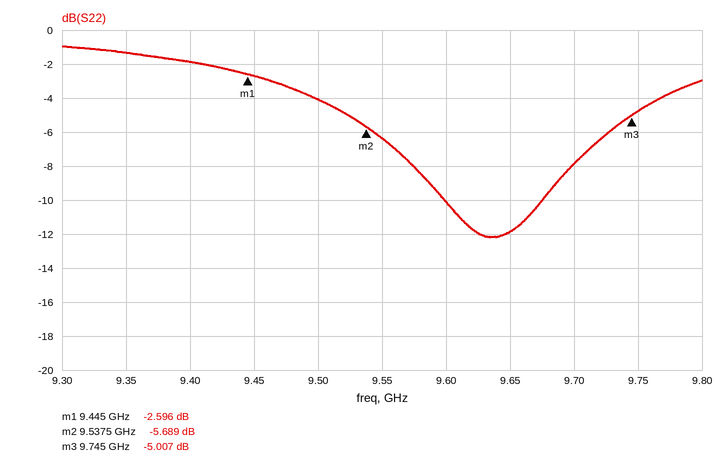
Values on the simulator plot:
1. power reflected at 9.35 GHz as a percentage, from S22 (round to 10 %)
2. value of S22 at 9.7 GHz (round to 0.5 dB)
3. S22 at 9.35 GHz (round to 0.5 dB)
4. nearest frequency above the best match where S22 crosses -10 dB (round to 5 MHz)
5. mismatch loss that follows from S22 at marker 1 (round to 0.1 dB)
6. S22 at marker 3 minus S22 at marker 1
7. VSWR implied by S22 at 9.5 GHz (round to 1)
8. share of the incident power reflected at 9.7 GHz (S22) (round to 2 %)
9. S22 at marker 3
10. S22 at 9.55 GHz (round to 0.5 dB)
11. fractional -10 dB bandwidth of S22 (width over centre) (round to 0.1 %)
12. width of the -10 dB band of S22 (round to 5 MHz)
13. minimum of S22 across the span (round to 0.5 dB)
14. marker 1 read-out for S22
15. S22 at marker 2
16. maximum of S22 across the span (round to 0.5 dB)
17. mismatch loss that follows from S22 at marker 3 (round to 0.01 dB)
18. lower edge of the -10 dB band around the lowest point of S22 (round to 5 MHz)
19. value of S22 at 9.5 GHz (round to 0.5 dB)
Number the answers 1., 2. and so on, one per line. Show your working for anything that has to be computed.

1. 10^(-1.5/10) ≈ 70.8 %, so 70 % to the nearest 10 %
2. -8.0 dB
3. -1.5 dB
4. 9.675 GHz
5. −10 log10(1 − 10^(-2.596/10)) ≈ 3.5 dB
6. -5.007 − (-2.596) = -2.411 dB
7. |Γ| = 10^(-4/20) = 0.6310; VSWR = (1 + 0.6310)/(1 − 0.6310) ≈ 4
8. 10^(-8/10) ≈ 16 %
9. -5.007 dB
10. -6.5 dB
11. 75 MHz / 9.6375 GHz ≈ 0.8 %
12. 9.675 GHz − 9.600 GHz = 75 MHz
13. -12.0 dB
14. -2.596 dB
15. -5.689 dB
16. -1.0 dB
17. −10 log10(1 − 10^(-5.007/10)) ≈ 1.65 dB
18. 9.600 GHz
19. -4.0 dB
